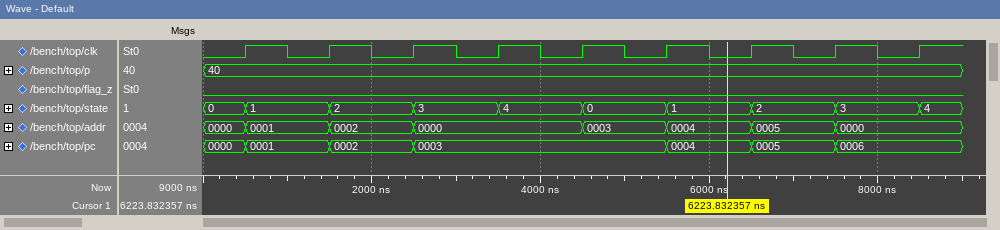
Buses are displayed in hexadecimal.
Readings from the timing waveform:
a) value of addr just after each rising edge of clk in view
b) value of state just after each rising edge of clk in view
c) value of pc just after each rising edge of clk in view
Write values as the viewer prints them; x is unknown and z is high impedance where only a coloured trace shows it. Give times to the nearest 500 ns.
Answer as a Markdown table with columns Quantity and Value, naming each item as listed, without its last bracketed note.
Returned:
| Quantity | Value |
|---|---|
| value of addr just after each rising edge of clk in view | 0001, 0002, 0000, 0000, 0003, 0004, 0005, 0000, 0000 |
| value of state just after each rising edge of clk in view | 1, 2, 3, 4, 0, 1, 2, 3, 4 |
| value of pc just after each rising edge of clk in view | 0001, 0002, 0003, 0003, 0003, 0004, 0005, 0006, 0006 |
